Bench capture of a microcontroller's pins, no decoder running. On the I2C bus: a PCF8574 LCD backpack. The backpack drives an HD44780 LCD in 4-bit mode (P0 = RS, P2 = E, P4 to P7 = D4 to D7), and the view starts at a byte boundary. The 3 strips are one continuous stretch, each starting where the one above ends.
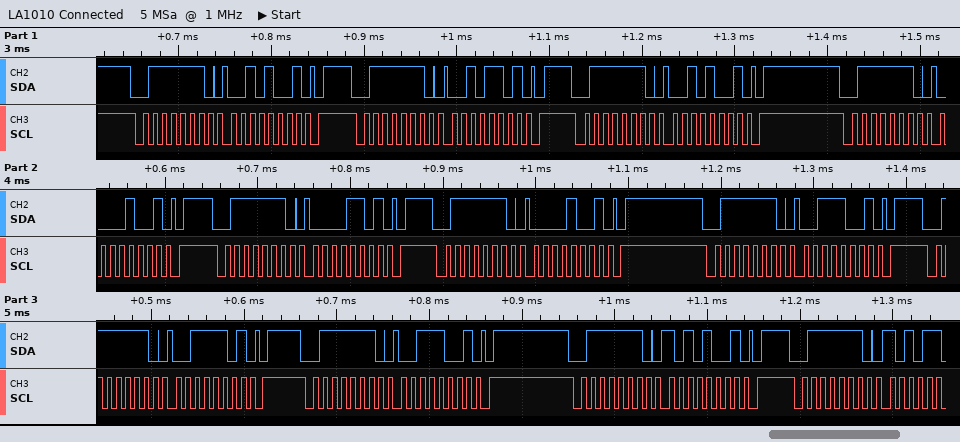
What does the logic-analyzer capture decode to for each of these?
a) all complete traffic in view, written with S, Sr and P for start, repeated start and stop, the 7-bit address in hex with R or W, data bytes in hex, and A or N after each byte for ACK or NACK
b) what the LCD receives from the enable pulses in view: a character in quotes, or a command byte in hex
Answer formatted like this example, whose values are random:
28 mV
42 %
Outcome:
S 3FW A 29 A P S 3FW A 2D A P S 3FW A 29 A P S 3FW A 09 A P S 3FW A 0D A P S 3FW A 09 A P S 3FW A 39 A P S 3FW A 3D A P S 3FW A 39 A P S 3FW A A9 A P S 3FW A
' '
